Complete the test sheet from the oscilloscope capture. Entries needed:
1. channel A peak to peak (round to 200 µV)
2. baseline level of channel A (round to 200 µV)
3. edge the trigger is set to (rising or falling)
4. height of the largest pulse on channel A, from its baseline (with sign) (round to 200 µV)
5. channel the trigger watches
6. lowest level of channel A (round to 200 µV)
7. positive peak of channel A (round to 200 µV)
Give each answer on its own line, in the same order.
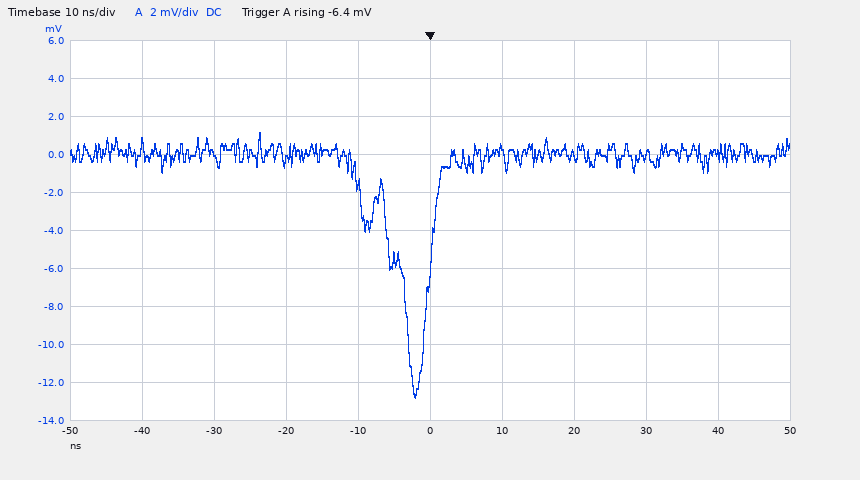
14.0 mV
0.0 mV
rising
-12.8 mV
channel A
-12.8 mV
1.2 mV
